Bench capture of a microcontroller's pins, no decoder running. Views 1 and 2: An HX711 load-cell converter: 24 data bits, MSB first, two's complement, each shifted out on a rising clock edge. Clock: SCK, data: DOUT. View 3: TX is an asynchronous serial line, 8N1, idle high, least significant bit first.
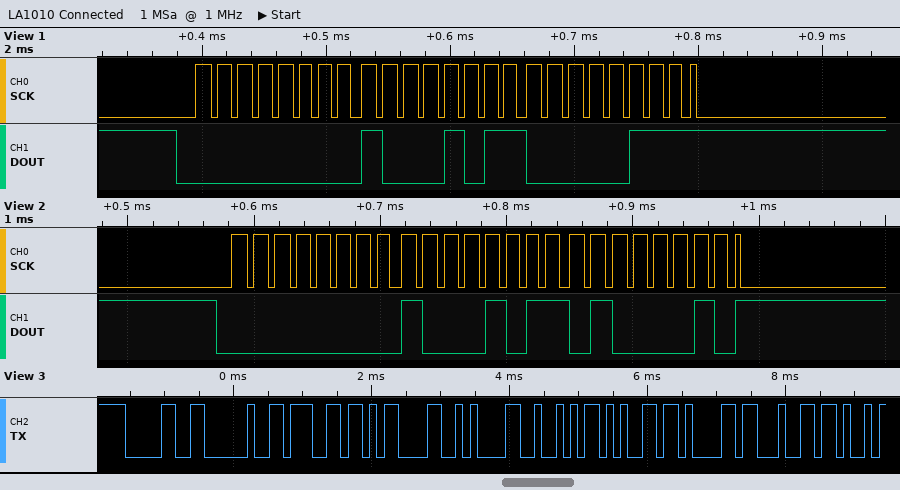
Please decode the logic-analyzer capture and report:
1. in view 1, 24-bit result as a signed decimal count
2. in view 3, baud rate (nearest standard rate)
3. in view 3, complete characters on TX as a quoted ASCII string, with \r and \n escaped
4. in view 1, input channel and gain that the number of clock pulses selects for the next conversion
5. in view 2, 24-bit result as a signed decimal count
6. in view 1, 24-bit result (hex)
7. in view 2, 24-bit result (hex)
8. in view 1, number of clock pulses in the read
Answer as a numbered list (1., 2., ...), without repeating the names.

1. 35591
2. 9600 baud
3. "0 g\r\nRead"
4. channel A, gain 128
5. 35650
6. 0x008B07
7. 0x008B42
8. 25
